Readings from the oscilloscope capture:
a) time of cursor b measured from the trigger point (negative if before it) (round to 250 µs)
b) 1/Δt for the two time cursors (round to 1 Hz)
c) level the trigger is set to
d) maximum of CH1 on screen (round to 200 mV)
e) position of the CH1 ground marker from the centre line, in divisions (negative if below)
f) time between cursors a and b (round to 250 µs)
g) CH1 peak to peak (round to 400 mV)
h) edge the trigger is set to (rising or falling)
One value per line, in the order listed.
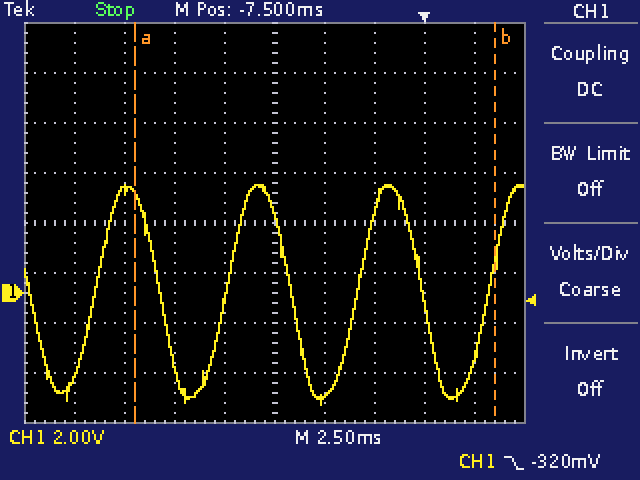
+3.50 ms
56 Hz
-320 mV
4.4 V
-1.4 div
18.00 ms
8.8 V
falling
